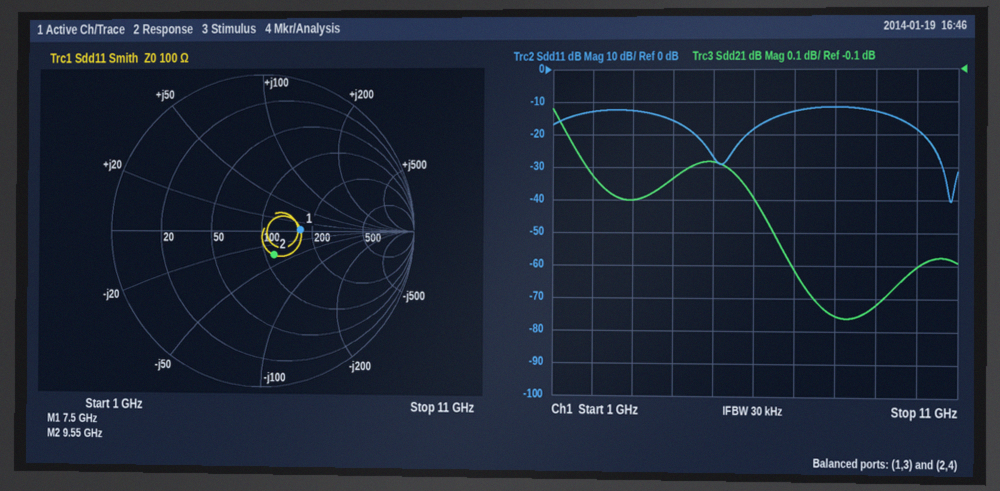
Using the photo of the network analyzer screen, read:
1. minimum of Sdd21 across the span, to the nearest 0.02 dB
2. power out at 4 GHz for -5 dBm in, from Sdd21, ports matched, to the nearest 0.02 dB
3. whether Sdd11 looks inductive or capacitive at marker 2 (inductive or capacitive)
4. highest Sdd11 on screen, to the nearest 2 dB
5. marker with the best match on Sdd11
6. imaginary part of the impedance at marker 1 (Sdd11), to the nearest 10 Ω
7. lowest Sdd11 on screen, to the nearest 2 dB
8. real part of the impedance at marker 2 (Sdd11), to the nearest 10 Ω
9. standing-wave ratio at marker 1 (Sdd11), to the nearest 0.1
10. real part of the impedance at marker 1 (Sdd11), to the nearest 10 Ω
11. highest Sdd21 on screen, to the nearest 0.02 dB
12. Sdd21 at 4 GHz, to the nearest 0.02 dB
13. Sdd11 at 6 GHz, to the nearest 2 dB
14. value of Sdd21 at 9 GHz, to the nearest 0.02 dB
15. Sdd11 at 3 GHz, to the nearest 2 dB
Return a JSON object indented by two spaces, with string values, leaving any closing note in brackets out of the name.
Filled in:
{
  "minimum of Sdd21 across the span, to the nearest 0.02 dB": "-0.86 dB",
  "power out at 4 GHz for -5 dBm in, from Sdd21, ports matched, to the nearest 0.02 dB": "-5.44 dBm",
  "whether Sdd11 looks inductive or capacitive at marker 2": "capacitive",
  "highest Sdd11 on screen, to the nearest 2 dB": "-12 dB",
  "marker with the best match on Sdd11": "marker 2",
  "imaginary part of the impedance at marker 1 (Sdd11), to the nearest 10 Ω": "0 Ω",
  "lowest Sdd11 on screen, to the nearest 2 dB": "-40 dB",
  "real part of the impedance at marker 2 (Sdd11), to the nearest 10 Ω": "110 Ω",
  "standing-wave ratio at marker 1 (Sdd11), to the nearest 0.1": "1.7",
  "real part of the impedance at marker 1 (Sdd11), to the nearest 10 Ω": "170 Ω",
  "highest Sdd21 on screen, to the nearest 0.02 dB": "-0.22 dB",
  "Sdd21 at 4 GHz, to the nearest 0.02 dB": "-0.44 dB",
  "Sdd11 at 6 GHz, to the nearest 2 dB": "-18 dB",
  "value of Sdd21 at 9 GHz, to the nearest 0.02 dB": "-0.82 dB",
  "Sdd11 at 3 GHz, to the nearest 2 dB": "-12 dB"
}
